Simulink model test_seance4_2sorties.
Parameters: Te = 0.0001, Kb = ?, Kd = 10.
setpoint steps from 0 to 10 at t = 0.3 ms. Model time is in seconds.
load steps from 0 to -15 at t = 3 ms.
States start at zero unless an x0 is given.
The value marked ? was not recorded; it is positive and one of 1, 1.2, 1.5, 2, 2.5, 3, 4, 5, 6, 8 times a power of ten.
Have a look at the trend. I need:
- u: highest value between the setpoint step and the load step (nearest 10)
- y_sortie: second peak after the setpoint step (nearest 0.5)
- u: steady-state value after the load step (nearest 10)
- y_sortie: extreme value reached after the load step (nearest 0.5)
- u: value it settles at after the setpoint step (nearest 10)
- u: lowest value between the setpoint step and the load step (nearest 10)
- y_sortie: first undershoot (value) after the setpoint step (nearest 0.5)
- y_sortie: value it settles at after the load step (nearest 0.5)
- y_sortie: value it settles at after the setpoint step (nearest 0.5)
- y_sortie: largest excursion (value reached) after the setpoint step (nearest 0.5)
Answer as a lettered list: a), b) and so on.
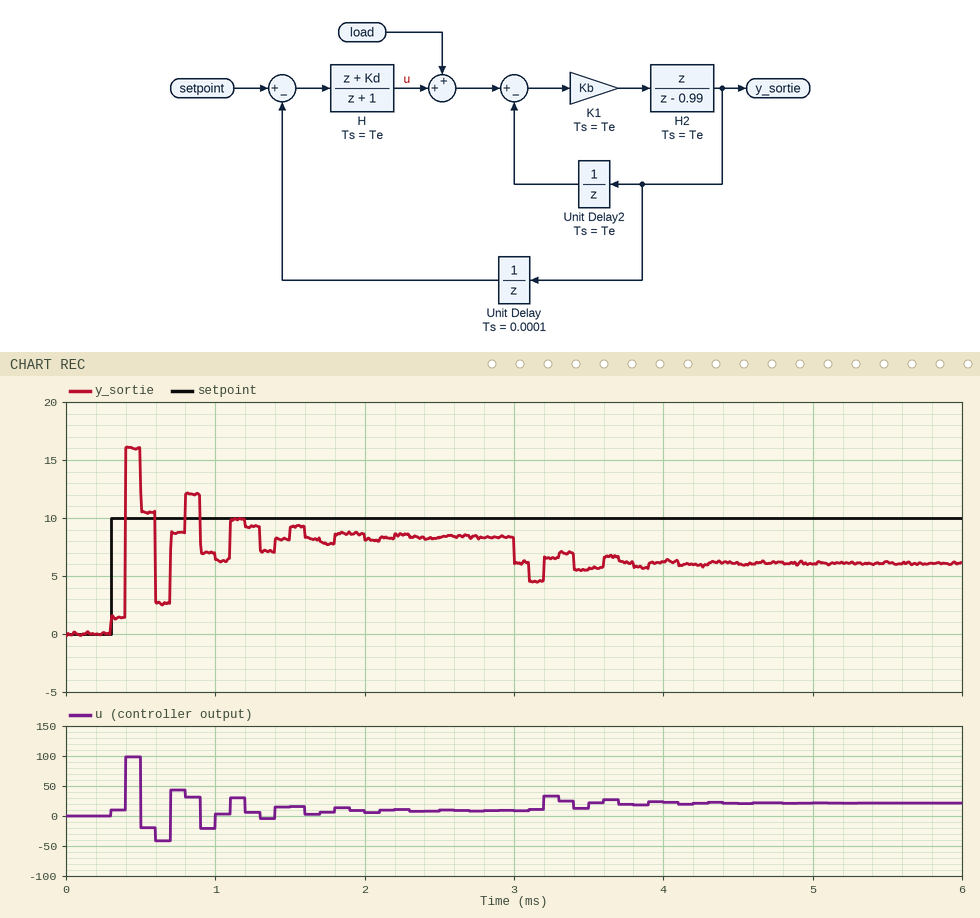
a) 100
b) 12.0
c) 20
d) 4.5
e) 10
f) -40
g) 2.5
h) 6.0
i) 8.5
j) 16.0
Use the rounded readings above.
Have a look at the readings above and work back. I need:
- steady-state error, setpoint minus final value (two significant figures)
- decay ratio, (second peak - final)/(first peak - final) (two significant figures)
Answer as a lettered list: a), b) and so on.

a) 1.5
b) 0.47
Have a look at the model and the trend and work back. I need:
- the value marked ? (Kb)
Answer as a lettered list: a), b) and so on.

a) 0.15
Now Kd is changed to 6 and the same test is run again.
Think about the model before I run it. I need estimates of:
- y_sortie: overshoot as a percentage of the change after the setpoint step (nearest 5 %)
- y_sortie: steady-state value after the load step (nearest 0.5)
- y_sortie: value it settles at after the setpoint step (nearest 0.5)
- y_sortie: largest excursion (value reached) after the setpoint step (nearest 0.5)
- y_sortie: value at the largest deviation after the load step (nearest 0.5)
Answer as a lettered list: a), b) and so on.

a) 30 %
b) 4.5
c) 7.5
d) 10.0
e) 4.0
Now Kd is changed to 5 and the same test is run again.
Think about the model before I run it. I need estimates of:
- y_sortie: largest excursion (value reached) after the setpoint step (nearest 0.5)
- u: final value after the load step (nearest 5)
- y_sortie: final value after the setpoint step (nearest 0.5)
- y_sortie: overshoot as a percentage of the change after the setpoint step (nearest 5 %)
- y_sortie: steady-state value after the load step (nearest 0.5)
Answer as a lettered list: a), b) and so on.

a) 8.5
b) 20
c) 7.5
d) 15 %
e) 3.5
